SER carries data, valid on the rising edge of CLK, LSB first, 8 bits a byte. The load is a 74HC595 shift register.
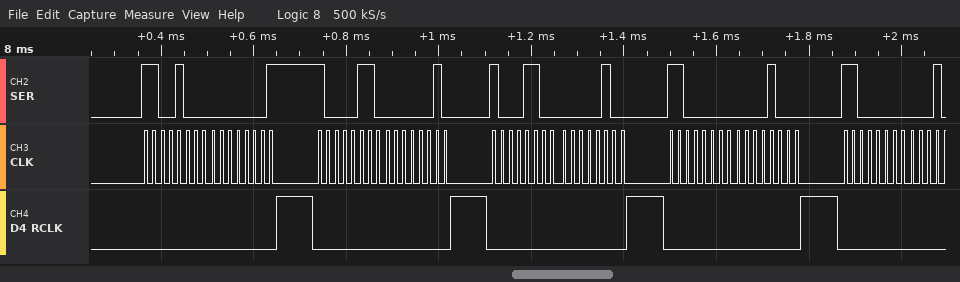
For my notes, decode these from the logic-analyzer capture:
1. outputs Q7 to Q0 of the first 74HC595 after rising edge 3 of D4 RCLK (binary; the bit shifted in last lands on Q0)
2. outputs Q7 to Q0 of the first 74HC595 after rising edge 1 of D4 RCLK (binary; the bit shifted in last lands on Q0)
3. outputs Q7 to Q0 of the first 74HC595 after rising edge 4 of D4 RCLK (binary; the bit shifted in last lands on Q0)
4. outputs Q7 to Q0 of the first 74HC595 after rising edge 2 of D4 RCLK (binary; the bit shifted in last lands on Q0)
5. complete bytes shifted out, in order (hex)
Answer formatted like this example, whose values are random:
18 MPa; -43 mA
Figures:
00000100; 00000001; 00001000; 00000010; 13 80 61 40 31 20 03 10 03
